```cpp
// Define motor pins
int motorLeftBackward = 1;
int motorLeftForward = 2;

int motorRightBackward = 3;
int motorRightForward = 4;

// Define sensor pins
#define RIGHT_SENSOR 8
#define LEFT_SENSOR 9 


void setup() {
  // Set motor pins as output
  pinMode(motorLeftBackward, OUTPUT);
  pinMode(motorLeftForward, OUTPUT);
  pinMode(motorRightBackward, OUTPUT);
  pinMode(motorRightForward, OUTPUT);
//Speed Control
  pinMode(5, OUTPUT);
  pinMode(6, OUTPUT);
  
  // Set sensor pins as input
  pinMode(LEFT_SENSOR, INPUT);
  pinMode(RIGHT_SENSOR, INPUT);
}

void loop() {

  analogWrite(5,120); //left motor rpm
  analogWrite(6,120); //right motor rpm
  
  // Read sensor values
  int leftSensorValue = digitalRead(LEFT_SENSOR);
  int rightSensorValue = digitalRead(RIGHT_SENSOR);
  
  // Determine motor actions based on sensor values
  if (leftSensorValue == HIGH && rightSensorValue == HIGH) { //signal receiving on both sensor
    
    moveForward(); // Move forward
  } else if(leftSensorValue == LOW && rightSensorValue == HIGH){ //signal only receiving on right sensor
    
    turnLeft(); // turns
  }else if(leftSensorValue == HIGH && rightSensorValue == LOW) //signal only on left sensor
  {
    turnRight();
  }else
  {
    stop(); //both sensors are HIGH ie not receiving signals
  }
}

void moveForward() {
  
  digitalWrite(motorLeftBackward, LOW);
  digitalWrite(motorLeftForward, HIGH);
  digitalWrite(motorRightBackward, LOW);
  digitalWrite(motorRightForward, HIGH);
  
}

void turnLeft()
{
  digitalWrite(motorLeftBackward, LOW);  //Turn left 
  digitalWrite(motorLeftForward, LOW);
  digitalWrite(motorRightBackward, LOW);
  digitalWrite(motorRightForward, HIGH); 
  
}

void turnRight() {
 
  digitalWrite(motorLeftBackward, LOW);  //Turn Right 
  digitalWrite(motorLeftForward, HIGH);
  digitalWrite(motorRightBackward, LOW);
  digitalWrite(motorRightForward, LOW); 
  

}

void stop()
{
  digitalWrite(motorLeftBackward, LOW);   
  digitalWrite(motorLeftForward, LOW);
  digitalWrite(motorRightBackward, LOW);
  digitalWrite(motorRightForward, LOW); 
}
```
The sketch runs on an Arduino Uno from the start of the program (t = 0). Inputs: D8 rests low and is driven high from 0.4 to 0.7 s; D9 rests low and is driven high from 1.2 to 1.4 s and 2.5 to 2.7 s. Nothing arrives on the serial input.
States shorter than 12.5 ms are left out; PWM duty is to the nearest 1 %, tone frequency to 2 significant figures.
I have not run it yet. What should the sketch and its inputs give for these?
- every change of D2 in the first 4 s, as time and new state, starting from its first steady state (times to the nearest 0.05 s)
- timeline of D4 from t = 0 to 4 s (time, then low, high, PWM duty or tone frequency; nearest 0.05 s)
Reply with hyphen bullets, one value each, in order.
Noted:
- 0 s low; 1.2 s high; 1.4 s low; 2.5 s high; 2.7 s low
- 0 s low; 0.4 s high; 0.7 s low
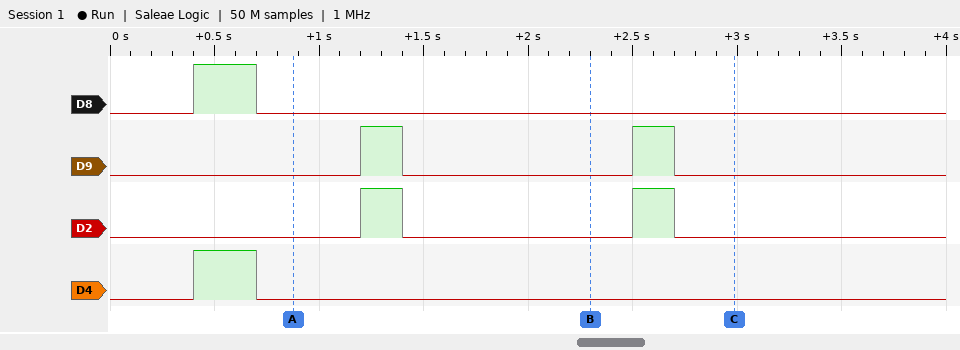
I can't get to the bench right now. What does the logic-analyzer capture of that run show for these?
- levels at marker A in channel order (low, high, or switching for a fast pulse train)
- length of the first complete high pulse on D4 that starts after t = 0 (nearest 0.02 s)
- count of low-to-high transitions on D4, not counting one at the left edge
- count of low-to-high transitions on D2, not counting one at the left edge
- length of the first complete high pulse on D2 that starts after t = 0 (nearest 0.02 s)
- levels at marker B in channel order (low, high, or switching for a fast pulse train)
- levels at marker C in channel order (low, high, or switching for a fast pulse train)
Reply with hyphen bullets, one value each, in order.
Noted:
- D8 low, D9 low, D2 low, D4 low
- 0.30 s
- 1
- 2
- 0.20 s
- D8 low, D9 low, D2 low, D4 low
- D8 low, D9 low, D2 low, D4 low
